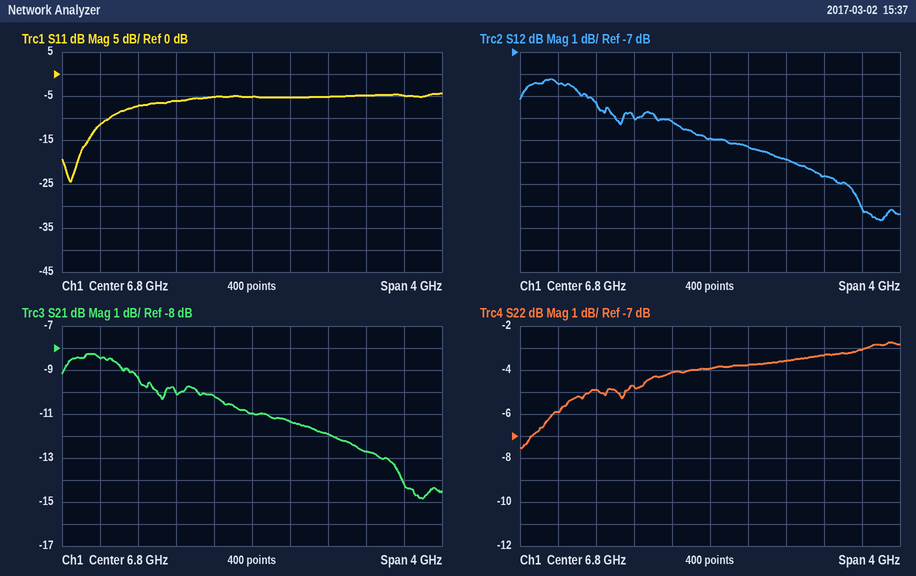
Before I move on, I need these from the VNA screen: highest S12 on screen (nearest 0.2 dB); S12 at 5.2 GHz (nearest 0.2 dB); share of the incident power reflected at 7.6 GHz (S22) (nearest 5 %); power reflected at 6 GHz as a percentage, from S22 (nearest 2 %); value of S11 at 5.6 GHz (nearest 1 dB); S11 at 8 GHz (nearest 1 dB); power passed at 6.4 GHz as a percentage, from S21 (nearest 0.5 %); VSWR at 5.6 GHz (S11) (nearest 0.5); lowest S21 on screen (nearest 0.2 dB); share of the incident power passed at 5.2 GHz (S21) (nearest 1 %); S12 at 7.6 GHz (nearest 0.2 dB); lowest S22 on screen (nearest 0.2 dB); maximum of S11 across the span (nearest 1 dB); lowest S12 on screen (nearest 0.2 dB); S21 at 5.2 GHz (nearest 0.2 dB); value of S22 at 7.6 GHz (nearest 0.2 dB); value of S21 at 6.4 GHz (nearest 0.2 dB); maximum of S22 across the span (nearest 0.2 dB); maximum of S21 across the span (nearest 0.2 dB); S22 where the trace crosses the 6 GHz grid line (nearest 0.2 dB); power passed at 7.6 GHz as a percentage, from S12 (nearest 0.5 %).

-8.2 dB
-8.4 dB
45 %
34 %
-7 dB
-5 dB
9.5 %
2.5
-14.8 dB
14 %
-11.8 dB
-7.6 dB
-4 dB
-14.6 dB
-8.4 dB
-3.6 dB
-10.2 dB
-2.8 dB
-8.2 dB
-4.8 dB
6.5 %
